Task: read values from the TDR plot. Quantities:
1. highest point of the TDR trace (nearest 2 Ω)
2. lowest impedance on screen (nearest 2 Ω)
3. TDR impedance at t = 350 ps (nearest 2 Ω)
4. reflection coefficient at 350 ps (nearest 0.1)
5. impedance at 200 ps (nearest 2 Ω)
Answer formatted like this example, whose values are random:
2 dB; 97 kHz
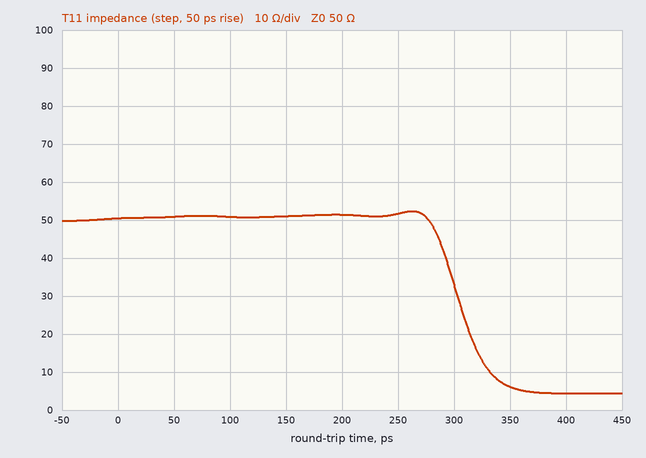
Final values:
52 Ω; 4 Ω; 6 Ω; -0.8; 52 Ω
